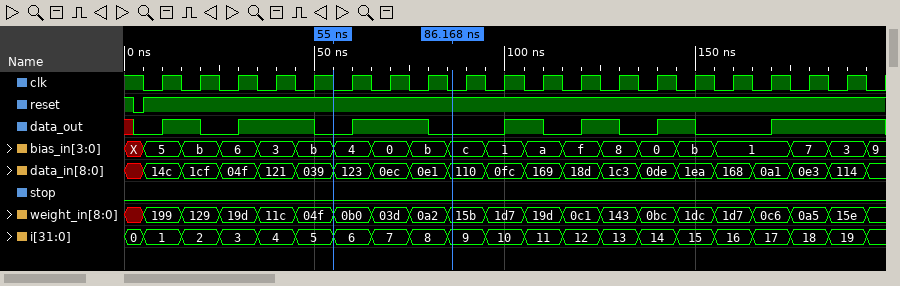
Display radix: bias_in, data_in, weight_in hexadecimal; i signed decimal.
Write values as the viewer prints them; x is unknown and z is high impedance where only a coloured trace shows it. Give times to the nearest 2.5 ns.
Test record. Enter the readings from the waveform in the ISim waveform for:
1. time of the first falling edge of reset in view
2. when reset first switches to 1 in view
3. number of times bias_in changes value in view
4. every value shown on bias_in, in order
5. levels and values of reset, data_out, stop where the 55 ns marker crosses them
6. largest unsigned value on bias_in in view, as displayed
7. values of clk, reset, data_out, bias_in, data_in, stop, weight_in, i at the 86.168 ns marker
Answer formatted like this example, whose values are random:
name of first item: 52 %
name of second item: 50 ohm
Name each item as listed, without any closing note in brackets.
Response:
time of the first falling edge of reset in view: 2.5 ns
when reset first switches to 1 in view: 5 ns
number of times bias_in changes value in view: 19
every value shown on bias_in, in order: X, 5, b, 6, 3, b, 4, 0, b, c, 1, a, f, 8, 0, b, 1, 7, 3, 9
levels and values of reset, data_out, stop where the 55 ns marker crosses them: reset=1, data_out=0, stop=0
largest unsigned value on bias_in in view, as displayed: f
values of clk, reset, data_out, bias_in, data_in, stop, weight_in, i at the 86.168 ns marker: clk=0, reset=1, data_out=0, bias_in=c, data_in=110, stop=0, weight_in=15b, i=9
